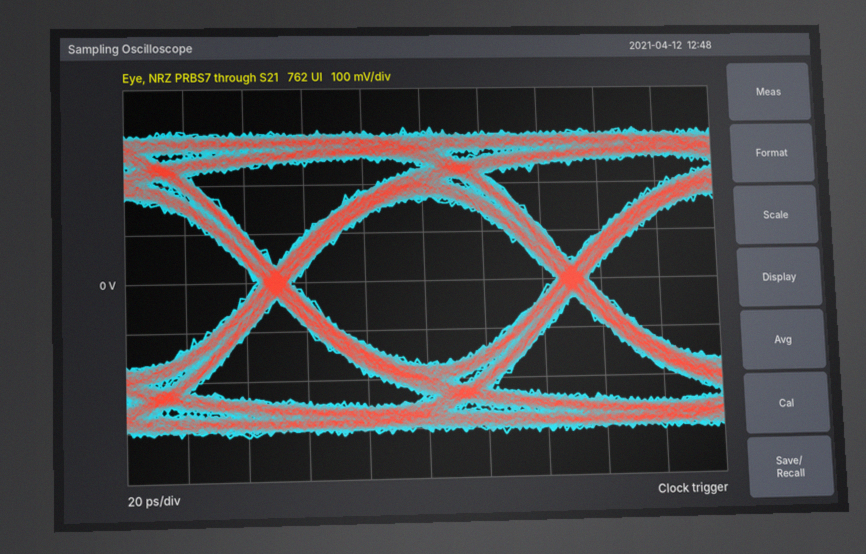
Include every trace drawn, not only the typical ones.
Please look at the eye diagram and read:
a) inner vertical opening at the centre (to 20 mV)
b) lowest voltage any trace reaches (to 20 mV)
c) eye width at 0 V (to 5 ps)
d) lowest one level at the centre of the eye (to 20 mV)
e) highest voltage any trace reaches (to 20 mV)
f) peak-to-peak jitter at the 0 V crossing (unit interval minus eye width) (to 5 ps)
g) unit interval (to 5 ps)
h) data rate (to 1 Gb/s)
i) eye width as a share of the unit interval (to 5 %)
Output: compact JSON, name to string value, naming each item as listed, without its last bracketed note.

{"inner vertical opening at the centre": "340 mV", "lowest voltage any trace reaches": "-320 mV", "eye width at 0 V": "90 ps", "lowest one level at the centre of the eye": "160 mV", "highest voltage any trace reaches": "320 mV", "peak-to-peak jitter at the 0 V crossing (unit interval minus eye width)": "10 ps", "unit interval": "100 ps", "data rate": "10 Gb/s", "eye width as a share of the unit interval": "90 %"}
